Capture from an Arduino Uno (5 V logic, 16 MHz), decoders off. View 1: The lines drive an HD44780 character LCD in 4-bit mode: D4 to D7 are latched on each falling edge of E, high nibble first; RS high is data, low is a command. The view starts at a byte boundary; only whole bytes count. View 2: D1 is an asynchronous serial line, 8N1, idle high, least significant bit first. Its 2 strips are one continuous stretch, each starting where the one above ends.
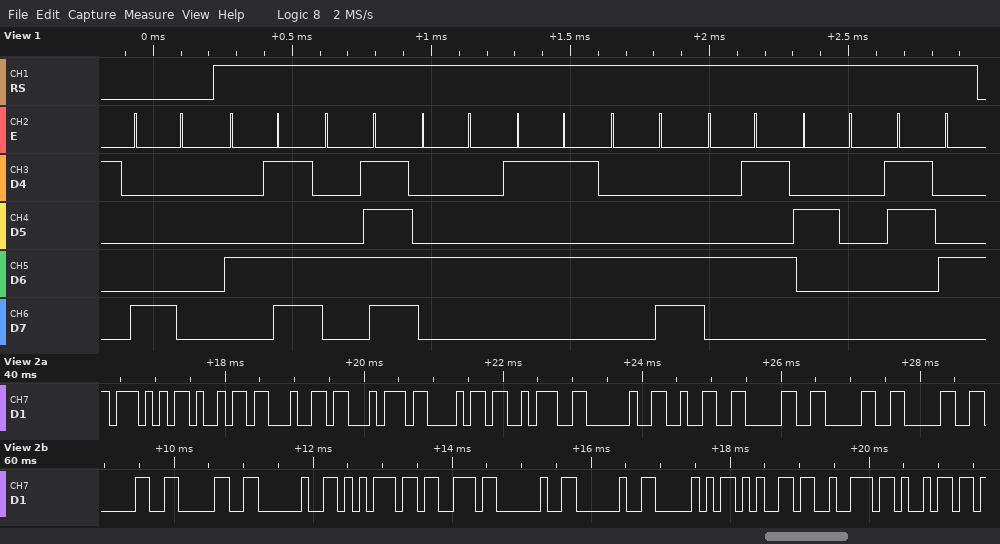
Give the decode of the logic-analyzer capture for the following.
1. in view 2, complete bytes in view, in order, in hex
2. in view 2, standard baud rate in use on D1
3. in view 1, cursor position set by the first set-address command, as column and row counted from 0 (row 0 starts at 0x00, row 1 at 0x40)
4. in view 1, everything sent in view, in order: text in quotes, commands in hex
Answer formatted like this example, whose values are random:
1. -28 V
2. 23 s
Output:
1. 57 69 64 74 68 3A 20 32 30 30 30 30 30 20 75 73 20 20 50 65 72 69
2. 9600 baud
3. column 0, row 0
4. 0x80 "MODULE 4"
